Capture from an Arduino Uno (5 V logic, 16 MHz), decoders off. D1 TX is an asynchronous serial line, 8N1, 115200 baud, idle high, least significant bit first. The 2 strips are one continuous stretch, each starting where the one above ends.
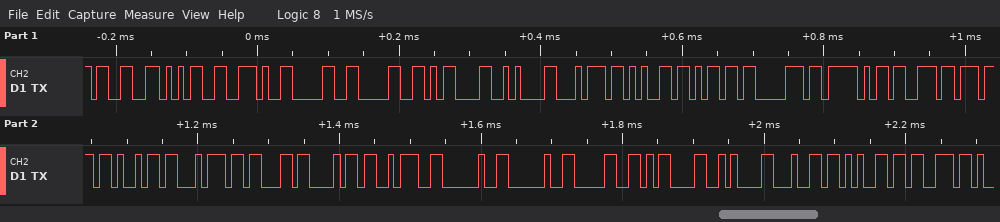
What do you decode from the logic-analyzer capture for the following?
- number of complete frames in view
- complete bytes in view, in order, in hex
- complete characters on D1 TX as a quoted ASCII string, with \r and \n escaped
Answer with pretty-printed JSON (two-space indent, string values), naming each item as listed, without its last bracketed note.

{
  "number of complete frames in view": "27",
  "complete bytes in view, in order, in hex": "33 35 2E 30 30 0D 0A 74 65 6D 70 5F 73 77 69 74 63 68 3A 20 20 30 0D 0A 64 65 73",
  "complete characters on D1 TX as a quoted ASCII string, with \\r and \\n escaped": "\"35.00\\r\\ntemp_switch:  0\\r\\ndes\""
}
